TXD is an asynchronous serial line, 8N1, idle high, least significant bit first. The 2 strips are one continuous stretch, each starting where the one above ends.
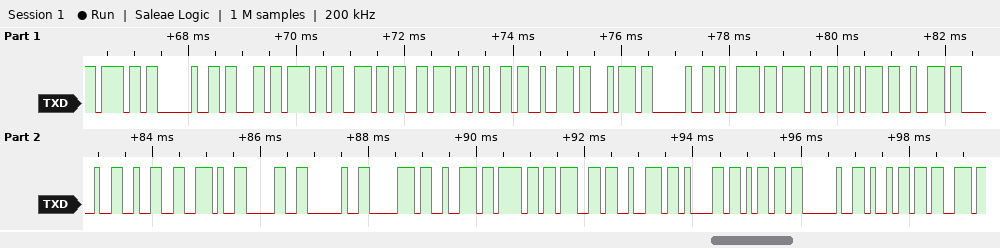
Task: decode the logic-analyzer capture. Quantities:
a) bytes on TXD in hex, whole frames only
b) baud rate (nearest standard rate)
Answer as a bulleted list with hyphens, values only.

- 6F 20 63 6F 6E 76 65 72 74 20 79 6F 75 72 20 32 2E 30 20 70 72 6F 67 72 61 6D 20 69 73
- 9600 baud
